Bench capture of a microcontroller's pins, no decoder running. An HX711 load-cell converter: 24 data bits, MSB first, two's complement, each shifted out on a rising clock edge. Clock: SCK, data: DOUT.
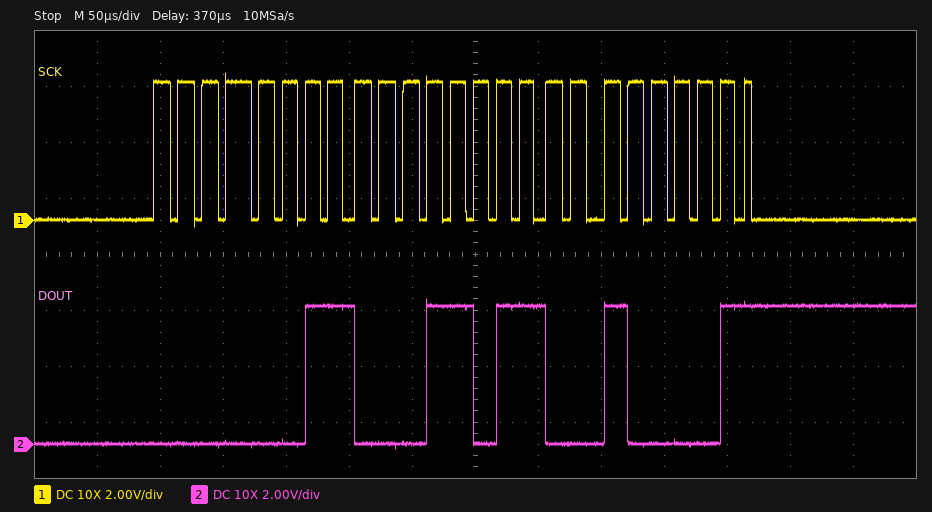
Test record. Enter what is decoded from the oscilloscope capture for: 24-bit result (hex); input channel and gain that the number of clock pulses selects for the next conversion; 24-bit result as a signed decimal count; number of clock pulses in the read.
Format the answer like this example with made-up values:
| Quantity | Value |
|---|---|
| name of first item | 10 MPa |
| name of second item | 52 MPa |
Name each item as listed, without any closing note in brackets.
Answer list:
| Quantity | Value |
|---|---|
| 24-bit result | 0x031B21 |
| input channel and gain that the number of clock pulses selects for the next conversion | channel A, gain 128 |
| 24-bit result as a signed decimal count | 203553 |
| number of clock pulses in the read | 25 |
